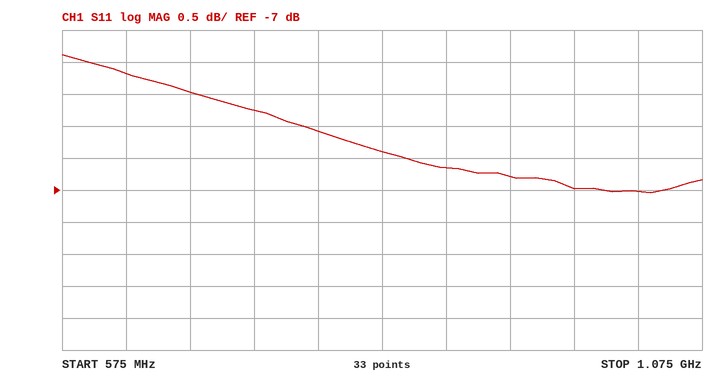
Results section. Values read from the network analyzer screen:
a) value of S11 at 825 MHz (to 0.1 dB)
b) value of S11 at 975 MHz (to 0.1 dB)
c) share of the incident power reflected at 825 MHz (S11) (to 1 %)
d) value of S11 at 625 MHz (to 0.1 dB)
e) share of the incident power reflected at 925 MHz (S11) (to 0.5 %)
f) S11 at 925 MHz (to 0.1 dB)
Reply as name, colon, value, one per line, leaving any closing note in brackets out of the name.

value of S11 at 825 MHz: -6.4 dB
value of S11 at 975 MHz: -7.0 dB
share of the incident power reflected at 825 MHz (S11): 23 %
value of S11 at 625 MHz: -5.2 dB
share of the incident power reflected at 925 MHz (S11): 21.0 %
S11 at 925 MHz: -6.8 dB
